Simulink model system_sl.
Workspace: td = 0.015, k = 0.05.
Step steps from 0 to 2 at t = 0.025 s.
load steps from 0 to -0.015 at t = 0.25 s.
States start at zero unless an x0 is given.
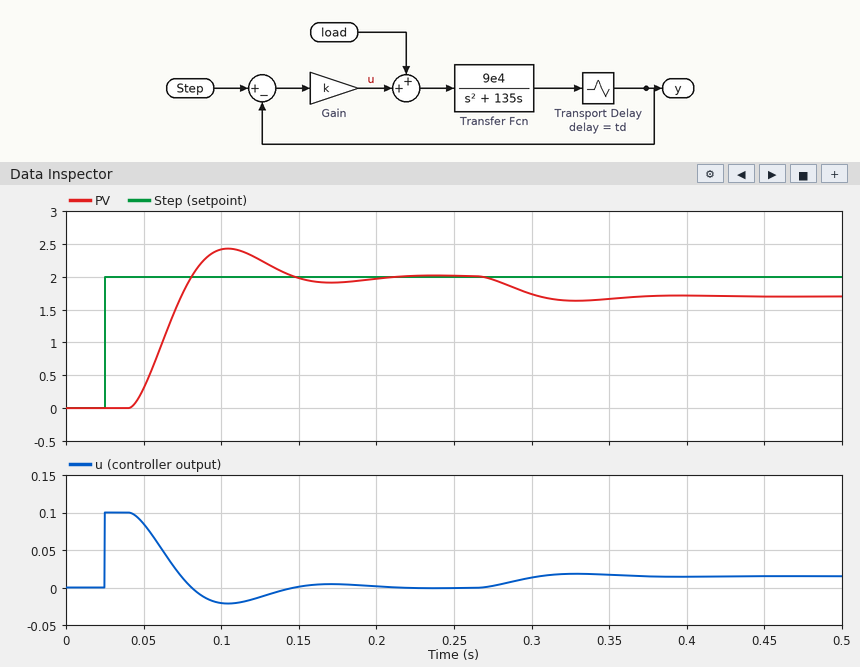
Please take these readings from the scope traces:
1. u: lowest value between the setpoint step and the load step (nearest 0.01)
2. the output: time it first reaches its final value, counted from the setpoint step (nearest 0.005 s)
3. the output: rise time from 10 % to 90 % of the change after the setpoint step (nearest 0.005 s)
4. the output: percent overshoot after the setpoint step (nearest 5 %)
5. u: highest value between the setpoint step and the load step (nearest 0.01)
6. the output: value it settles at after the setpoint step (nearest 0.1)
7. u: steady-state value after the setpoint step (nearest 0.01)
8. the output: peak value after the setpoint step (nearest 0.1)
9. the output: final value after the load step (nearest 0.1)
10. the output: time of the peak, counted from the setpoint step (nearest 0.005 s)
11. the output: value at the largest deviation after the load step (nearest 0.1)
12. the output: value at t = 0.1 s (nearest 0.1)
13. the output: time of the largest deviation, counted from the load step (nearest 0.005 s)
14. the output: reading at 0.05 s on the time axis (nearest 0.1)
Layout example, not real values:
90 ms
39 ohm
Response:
-0.02
0.055 s
0.030 s
20 %
0.10
2.0
0.00
2.4
1.7
0.080 s
1.6
2.4
0.080 s
0.3
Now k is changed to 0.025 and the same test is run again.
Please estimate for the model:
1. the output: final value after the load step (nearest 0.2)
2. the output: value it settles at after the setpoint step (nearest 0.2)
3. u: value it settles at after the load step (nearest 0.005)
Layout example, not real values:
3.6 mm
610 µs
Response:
1.4
2.0
0.015
